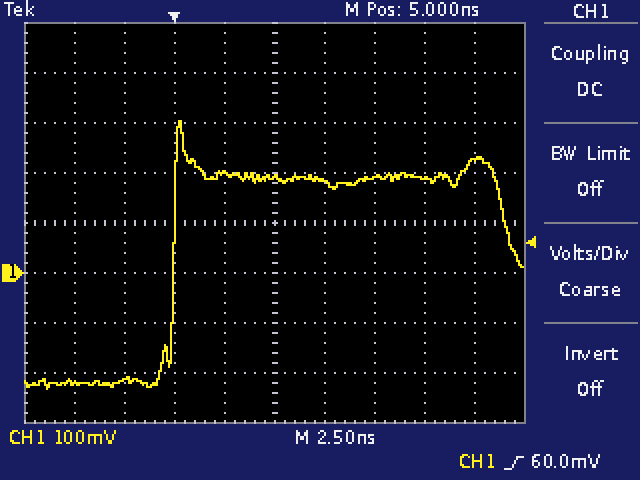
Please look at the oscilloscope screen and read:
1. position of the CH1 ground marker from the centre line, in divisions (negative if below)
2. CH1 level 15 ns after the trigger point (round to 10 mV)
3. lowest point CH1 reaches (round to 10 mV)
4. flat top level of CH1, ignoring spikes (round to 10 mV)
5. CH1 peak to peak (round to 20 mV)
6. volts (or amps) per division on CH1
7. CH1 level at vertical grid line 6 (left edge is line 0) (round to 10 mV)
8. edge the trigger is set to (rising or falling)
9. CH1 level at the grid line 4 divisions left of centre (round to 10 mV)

-1.0 div
230 mV
-230 mV
190 mV
540 mV
100 mV
180 mV
rising
-220 mV
